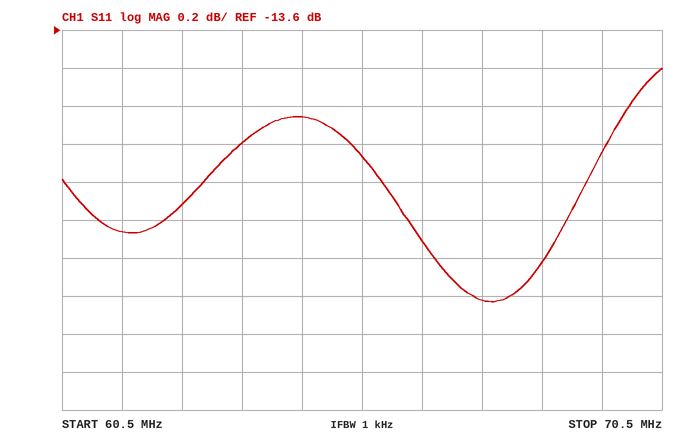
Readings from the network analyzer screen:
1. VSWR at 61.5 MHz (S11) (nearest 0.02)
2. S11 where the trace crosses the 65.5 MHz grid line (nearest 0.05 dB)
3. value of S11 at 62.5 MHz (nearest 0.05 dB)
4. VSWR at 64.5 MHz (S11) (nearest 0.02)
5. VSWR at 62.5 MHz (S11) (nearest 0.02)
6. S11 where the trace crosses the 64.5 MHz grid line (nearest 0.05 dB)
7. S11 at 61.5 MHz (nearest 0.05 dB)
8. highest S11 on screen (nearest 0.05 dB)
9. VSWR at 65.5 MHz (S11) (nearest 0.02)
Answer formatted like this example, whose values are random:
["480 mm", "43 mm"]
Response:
["1.46", "-14.25 dB", "-14.50 dB", "1.50", "1.46", "-14.05 dB", "-14.65 dB", "-13.80 dB", "1.48"]
